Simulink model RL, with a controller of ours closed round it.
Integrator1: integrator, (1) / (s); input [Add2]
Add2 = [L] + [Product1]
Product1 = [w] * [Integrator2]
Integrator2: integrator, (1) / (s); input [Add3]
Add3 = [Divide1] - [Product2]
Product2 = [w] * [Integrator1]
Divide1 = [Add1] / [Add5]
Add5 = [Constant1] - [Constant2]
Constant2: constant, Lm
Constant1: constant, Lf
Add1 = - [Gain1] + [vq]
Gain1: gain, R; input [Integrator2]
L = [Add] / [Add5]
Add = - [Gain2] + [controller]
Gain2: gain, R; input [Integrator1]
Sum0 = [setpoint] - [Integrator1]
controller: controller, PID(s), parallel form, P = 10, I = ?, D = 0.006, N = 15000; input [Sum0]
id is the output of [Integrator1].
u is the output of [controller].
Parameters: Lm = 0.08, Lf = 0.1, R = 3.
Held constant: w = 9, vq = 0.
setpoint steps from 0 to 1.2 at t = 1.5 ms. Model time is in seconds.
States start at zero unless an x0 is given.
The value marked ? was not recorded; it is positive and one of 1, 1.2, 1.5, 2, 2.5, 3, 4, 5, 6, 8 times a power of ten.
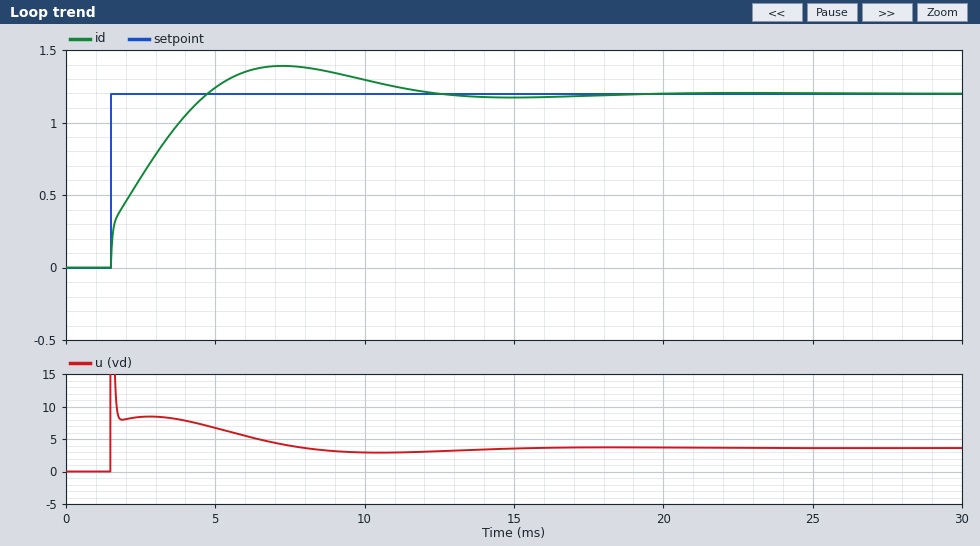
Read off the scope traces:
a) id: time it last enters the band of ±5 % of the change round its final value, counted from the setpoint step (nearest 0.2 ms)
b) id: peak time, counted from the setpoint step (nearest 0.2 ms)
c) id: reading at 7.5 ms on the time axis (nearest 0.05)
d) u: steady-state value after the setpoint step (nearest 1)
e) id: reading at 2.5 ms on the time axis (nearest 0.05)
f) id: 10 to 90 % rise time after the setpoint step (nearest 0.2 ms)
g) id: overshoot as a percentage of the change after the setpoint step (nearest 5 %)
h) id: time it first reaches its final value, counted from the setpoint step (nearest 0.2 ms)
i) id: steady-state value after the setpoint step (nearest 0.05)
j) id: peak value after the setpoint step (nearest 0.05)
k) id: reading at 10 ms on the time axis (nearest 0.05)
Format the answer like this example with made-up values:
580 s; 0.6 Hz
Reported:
9.2 ms; 5.8 ms; 1.40; 4; 0.60; 2.6 ms; 15 %; 3.2 ms; 1.20; 1.40; 1.30
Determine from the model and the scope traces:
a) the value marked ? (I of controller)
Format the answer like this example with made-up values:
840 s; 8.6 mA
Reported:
6000
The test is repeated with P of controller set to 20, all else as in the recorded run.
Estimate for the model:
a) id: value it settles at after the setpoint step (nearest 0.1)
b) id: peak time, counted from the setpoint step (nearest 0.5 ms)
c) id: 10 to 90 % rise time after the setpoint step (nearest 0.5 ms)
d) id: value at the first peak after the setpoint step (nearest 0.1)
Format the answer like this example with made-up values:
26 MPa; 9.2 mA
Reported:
1.2; 5.0 ms; 2.0 ms; 1.3
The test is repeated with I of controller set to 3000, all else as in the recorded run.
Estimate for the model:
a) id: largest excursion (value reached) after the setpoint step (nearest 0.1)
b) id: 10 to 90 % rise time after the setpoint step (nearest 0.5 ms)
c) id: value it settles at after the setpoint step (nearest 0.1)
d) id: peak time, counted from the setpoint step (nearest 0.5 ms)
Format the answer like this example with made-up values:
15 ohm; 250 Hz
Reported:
1.3; 3.5 ms; 1.2; 8.5 ms
